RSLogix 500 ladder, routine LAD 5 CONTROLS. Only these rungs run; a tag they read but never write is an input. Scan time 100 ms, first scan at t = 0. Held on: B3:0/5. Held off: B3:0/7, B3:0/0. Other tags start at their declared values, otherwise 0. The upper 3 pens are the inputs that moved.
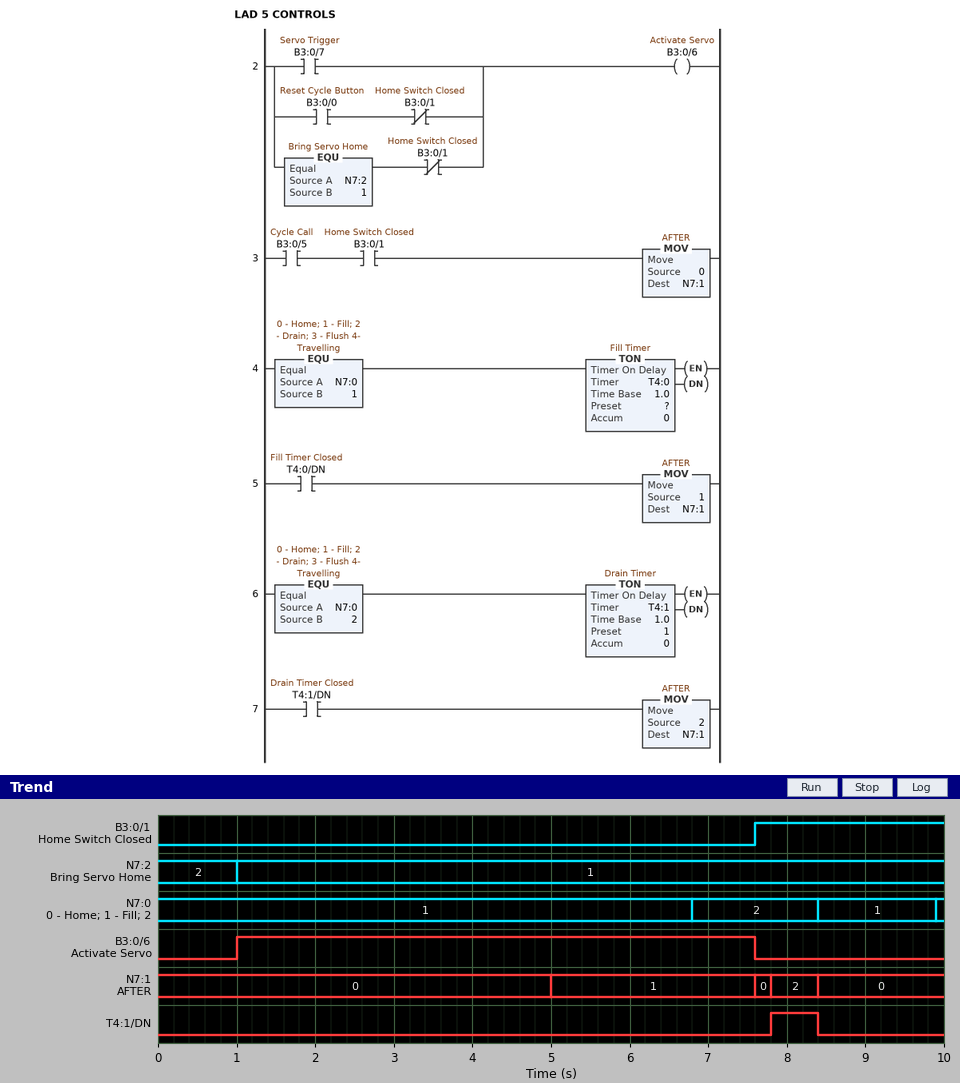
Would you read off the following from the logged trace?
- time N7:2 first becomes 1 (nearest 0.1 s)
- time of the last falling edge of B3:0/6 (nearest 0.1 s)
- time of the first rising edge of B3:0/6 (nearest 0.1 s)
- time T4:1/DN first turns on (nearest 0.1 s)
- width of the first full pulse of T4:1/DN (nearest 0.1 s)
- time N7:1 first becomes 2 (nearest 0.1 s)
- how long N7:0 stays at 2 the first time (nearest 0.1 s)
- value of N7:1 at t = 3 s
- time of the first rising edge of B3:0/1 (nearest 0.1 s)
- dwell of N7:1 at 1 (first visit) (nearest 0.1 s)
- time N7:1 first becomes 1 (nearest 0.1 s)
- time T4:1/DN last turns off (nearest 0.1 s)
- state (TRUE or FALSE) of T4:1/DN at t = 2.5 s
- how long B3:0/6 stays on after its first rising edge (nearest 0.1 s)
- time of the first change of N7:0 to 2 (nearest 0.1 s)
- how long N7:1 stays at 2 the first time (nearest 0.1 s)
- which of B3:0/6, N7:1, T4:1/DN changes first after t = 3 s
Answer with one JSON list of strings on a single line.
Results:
["1.0 s", "7.6 s", "1.0 s", "7.8 s", "0.6 s", "7.8 s", "1.6 s", "0", "7.6 s", "2.6 s", "5.0 s", "8.4 s", "FALSE", "6.6 s", "6.8 s", "0.6 s", "N7:1"]
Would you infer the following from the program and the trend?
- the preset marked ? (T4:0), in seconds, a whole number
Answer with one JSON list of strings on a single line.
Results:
["5 s"]
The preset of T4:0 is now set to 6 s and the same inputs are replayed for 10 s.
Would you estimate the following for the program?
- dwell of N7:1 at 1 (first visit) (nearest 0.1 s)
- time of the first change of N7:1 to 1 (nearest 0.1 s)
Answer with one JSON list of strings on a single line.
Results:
["1.6 s", "6.0 s"]
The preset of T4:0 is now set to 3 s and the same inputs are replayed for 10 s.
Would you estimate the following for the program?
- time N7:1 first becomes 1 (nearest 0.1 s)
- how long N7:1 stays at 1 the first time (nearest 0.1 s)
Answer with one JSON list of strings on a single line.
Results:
["3.0 s", "4.6 s"]
